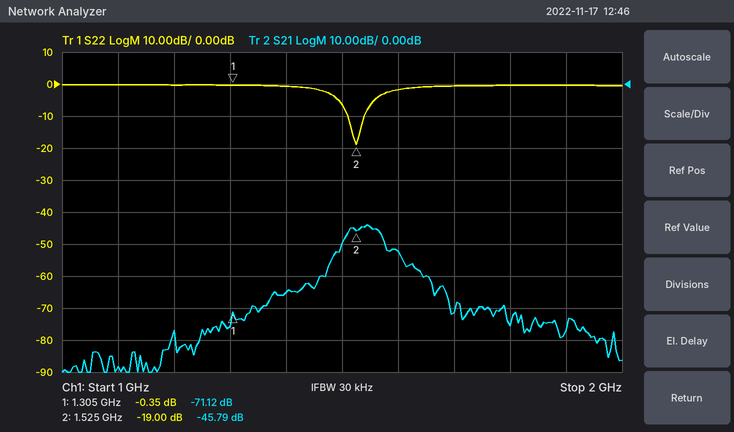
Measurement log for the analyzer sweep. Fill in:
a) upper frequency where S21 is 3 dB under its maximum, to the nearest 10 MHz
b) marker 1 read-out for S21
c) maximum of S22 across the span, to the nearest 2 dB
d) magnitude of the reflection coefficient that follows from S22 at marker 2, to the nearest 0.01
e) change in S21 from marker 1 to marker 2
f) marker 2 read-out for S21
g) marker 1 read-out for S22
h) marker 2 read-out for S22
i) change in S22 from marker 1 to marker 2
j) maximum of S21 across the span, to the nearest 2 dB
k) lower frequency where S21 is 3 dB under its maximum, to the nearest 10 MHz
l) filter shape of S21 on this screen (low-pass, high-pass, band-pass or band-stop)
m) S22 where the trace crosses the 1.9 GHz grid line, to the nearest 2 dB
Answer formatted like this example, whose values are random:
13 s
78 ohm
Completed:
1.57 GHz
-71.12 dB
0 dB
0.11
25.33 dB
-45.79 dB
-0.35 dB
-19.00 dB
-18.65 dB
-44 dB
1.51 GHz
band-pass
0 dB
